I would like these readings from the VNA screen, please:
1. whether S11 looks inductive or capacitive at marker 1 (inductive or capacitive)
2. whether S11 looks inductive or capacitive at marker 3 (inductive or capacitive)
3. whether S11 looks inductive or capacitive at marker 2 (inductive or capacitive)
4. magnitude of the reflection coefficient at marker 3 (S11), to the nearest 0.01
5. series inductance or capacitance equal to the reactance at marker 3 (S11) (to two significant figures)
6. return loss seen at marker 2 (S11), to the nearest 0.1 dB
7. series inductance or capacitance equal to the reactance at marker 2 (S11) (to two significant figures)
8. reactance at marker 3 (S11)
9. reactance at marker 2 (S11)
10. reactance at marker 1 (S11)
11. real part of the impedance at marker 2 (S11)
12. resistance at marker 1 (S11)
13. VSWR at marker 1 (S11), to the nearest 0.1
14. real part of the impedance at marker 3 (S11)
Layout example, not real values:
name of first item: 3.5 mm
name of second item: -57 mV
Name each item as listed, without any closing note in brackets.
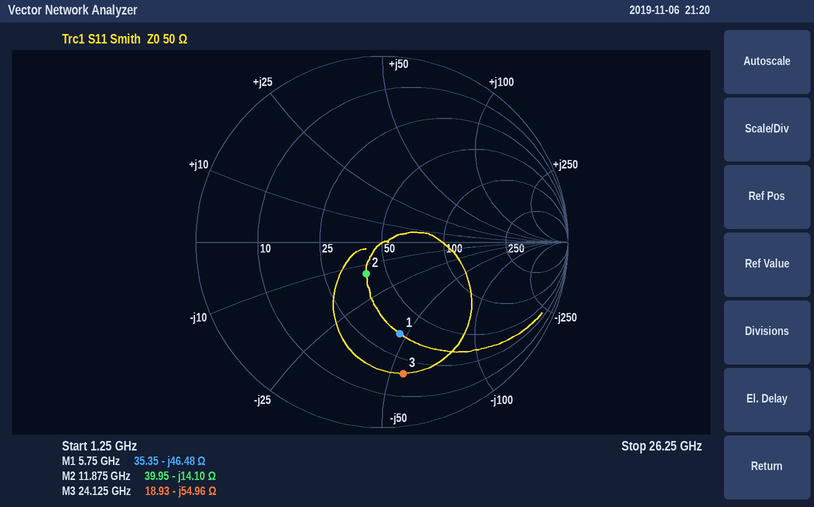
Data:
whether S11 looks inductive or capacitive at marker 1: capacitive
whether S11 looks inductive or capacitive at marker 3: capacitive
whether S11 looks inductive or capacitive at marker 2: capacitive
magnitude of the reflection coefficient at marker 3 (S11), to the nearest 0.01: 0.72
series inductance or capacitance equal to the reactance at marker 3 (S11): 120 fF
return loss seen at marker 2 (S11), to the nearest 0.1 dB: 14.4 dB
series inductance or capacitance equal to the reactance at marker 2 (S11): 950 fF
reactance at marker 3: -54.96 Ω
reactance at marker 2: -14.10 Ω
reactance at marker 1: -46.48 Ω
real part of the impedance at marker 2: 39.95 Ω
resistance at marker 1: 35.35 Ω
VSWR at marker 1 (S11), to the nearest 0.1: 3.0
real part of the impedance at marker 3: 18.93 Ω
